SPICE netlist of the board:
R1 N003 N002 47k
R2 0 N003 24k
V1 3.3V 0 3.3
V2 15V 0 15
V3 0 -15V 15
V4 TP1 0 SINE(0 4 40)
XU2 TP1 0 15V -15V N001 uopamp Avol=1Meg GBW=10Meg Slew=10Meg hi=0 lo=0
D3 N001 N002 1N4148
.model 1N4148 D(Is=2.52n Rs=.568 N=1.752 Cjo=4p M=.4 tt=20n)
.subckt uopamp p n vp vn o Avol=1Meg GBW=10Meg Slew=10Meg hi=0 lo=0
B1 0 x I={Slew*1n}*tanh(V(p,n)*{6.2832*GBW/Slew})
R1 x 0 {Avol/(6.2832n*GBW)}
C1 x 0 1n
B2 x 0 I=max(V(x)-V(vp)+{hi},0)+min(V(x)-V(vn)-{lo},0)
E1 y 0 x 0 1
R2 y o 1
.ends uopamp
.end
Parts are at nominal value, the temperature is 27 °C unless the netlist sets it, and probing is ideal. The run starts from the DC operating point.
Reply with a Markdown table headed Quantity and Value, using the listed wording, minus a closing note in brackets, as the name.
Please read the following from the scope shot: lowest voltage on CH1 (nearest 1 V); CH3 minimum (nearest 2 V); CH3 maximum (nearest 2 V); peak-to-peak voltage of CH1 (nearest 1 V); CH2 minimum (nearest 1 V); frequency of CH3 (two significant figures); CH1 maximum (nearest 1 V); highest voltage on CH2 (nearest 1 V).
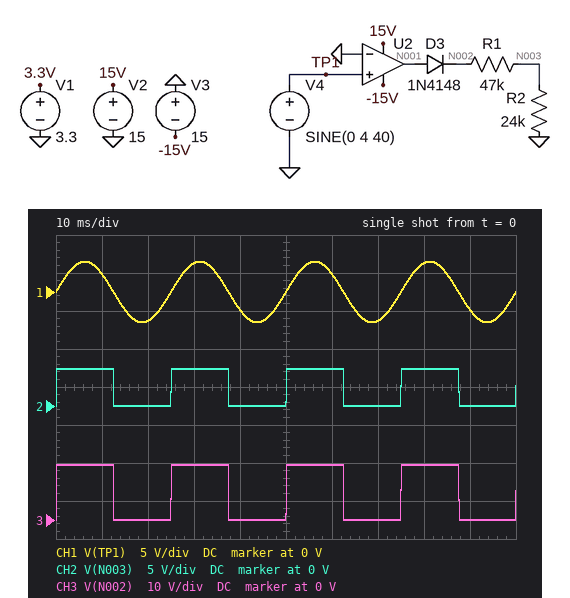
| Quantity | Value |
|---|---|
| lowest voltage on CH1 | -4 V |
| CH3 minimum | 0 V |
| CH3 maximum | 14 V |
| peak-to-peak voltage of CH1 | 8 V |
| CH2 minimum | 0 V |
| frequency of CH3 | 40 Hz |
| CH1 maximum | 4 V |
| highest voltage on CH2 | 5 V |
